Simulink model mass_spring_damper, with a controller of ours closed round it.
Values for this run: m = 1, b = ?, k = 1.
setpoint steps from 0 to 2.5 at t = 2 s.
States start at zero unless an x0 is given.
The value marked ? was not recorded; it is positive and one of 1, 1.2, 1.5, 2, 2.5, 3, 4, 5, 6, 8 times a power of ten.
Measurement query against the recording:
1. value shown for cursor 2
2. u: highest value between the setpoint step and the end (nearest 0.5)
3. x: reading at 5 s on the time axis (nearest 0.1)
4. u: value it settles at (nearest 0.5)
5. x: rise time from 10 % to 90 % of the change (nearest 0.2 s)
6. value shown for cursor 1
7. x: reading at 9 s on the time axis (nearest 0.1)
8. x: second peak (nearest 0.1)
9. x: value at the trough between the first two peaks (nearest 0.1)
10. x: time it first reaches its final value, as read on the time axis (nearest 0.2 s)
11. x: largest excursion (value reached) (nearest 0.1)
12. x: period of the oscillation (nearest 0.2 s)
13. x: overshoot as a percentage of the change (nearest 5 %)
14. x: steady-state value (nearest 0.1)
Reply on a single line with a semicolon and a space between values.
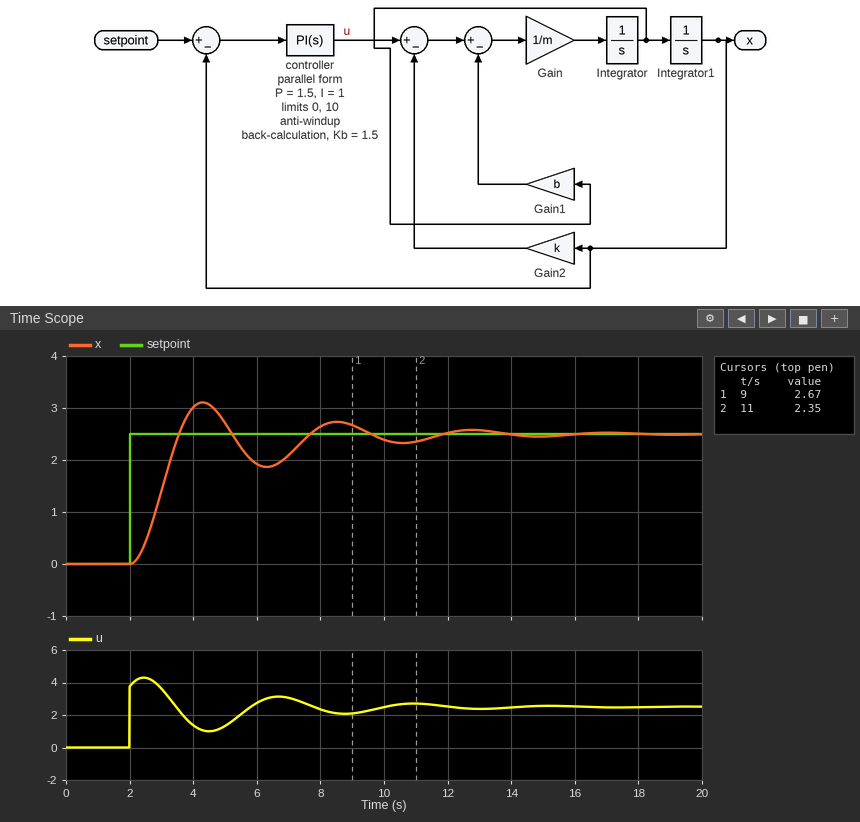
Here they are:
2.35; 4.5; 2.7; 2.5; 1.0 s; 2.67; 2.7; 2.7; 1.9; 3.6 s; 3.1; 4.2 s; 25 %; 2.5
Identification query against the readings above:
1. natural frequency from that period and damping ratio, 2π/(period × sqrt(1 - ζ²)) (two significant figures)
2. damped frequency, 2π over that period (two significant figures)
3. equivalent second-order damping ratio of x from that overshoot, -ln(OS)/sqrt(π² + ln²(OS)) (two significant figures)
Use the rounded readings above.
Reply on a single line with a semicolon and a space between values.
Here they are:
1.6 rad/s; 1.5 rad/s; 0.40
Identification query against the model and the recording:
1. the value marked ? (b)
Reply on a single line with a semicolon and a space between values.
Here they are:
1
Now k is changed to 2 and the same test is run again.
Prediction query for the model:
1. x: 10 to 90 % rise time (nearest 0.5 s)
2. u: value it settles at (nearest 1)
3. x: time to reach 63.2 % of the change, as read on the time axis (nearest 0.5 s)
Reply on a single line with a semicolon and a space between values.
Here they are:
1.5 s; 5; 3.0 s
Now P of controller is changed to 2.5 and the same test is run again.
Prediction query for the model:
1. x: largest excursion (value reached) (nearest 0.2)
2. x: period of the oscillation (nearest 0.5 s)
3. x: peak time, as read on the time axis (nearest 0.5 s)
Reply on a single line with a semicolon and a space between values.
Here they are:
3.2; 3.5 s; 4.0 s
